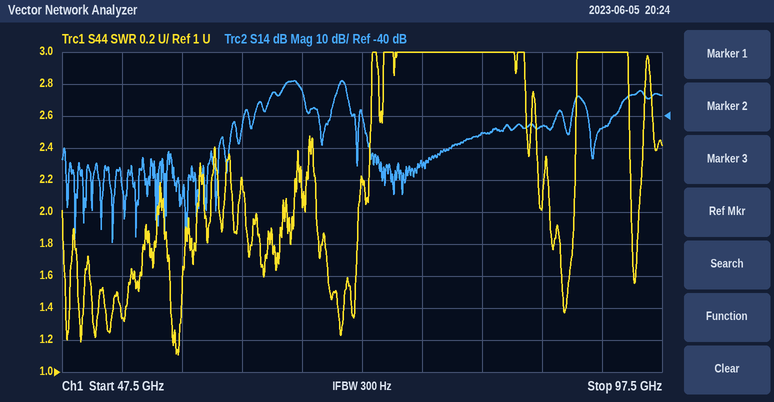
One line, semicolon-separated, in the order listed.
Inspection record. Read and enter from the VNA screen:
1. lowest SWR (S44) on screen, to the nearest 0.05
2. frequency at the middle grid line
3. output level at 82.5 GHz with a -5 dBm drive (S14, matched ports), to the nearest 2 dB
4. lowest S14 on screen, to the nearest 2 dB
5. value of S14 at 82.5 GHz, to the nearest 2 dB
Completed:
1.10; 72.5 GHz; -50 dBm; -80 dB; -46 dB
